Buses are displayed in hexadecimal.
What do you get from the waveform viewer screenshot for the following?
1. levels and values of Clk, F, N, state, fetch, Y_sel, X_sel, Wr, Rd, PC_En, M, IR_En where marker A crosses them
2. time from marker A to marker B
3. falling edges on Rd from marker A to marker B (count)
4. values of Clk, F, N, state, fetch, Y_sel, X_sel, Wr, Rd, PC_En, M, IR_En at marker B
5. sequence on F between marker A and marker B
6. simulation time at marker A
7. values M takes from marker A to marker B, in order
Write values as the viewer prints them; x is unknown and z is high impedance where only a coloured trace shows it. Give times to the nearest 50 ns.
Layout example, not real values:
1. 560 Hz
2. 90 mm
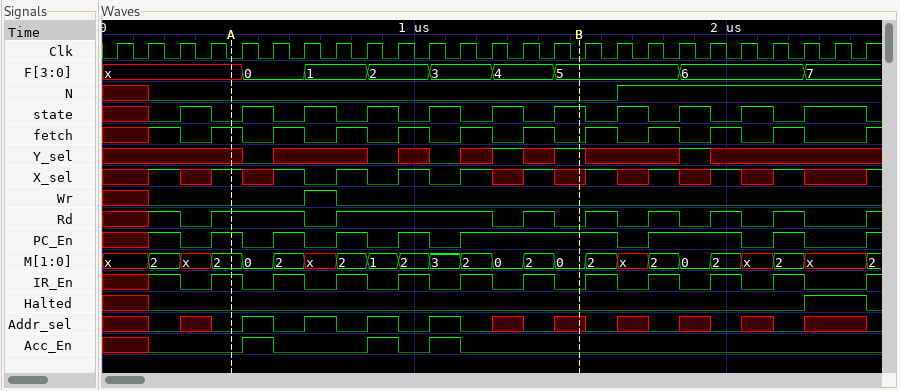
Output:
1. Clk=0, F=x, N=0, state=0, fetch=1, Y_sel=x, X_sel=1, Wr=0, Rd=1, PC_En=1, M=2, IR_En=1
2. 1100 ns
3. 3
4. Clk=0, F=5, N=0, state=1, fetch=0, Y_sel=1, X_sel=x, Wr=0, Rd=0, PC_En=1, M=0, IR_En=0
5. x, 0, 1, 2, 3, 4, 5
6. 400 ns
7. 2, 0, 2, x, 2, 1, 2, 3, 2, 0, 2, 0
